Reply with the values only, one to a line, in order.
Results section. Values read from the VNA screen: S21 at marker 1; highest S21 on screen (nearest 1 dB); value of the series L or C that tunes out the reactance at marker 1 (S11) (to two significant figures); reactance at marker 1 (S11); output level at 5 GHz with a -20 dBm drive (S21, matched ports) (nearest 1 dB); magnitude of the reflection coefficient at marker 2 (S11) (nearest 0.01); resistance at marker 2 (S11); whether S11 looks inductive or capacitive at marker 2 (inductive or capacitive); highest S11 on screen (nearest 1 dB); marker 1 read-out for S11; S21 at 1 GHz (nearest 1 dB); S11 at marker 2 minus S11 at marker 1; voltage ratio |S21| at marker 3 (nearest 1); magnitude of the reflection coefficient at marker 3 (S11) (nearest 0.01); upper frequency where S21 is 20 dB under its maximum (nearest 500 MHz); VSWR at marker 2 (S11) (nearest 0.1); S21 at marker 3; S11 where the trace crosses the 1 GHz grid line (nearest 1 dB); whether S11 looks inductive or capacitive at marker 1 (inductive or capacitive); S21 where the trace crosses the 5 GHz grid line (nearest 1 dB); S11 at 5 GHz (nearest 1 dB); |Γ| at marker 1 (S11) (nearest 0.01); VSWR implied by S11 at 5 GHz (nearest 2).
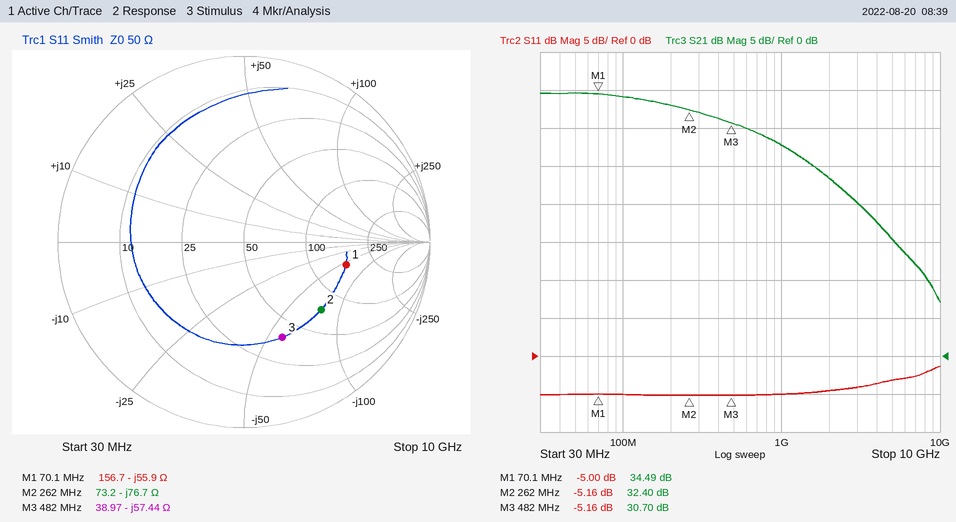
34.49 dB
35 dB
130 nH
-55.9 Ω
-5 dBm
0.55
73.2 Ω
capacitive
-1 dB
-5.00 dB
28 dB
-0.16 dB
34
0.55
5.5 GHz
3.5
30.70 dB
-5 dB
capacitive
15 dB
-3 dB
0.56
6
